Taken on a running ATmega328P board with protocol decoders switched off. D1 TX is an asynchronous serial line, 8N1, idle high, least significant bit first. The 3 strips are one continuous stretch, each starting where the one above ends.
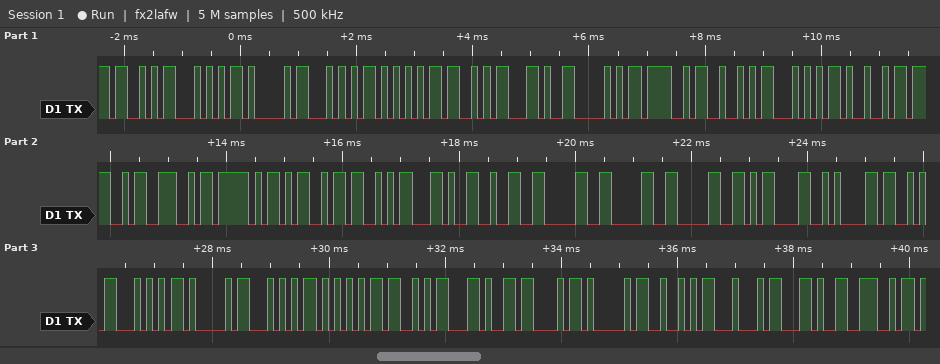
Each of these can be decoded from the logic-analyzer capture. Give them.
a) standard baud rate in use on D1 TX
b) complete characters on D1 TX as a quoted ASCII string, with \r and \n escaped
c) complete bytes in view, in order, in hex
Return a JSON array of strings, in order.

["9600 baud", "\"STATUS,PORTION_MS,2000\\r\\nSTATUS,CARD,N\"", "53 54 41 54 55 53 2C 50 4F 52 54 49 4F 4E 5F 4D 53 2C 32 30 30 30 0D 0A 53 54 41 54 55 53 2C 43 41 52 44 2C 4E"]
